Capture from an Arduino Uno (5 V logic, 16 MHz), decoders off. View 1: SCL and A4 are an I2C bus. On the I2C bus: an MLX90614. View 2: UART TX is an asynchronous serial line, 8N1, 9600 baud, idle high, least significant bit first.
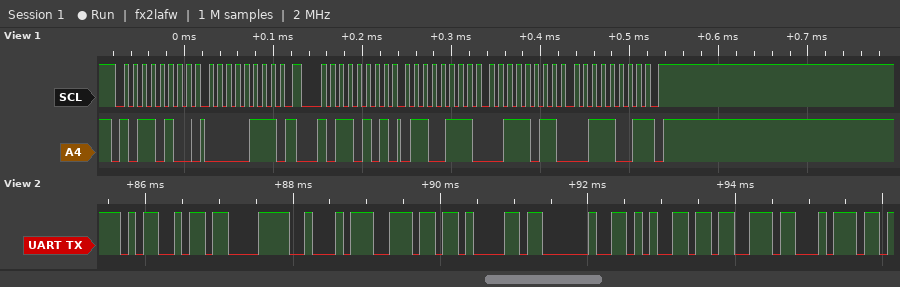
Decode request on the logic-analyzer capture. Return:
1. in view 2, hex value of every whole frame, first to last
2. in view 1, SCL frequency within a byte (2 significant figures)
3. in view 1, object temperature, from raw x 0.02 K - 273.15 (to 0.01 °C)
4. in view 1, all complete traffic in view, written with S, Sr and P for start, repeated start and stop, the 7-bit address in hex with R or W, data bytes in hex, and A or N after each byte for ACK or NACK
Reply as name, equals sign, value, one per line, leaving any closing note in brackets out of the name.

in view 2, hex value of every whole frame, first to last = 4D C3 A2 6E 61 20 65 73 74
in view 1, SCL frequency within a byte = 100 kHz
in view 1, object temperature, from raw x 0.02 K - 273.15 = 30.99 °C
in view 1, all complete traffic in view, written with S, Sr and P for start, repeated start and stop, the 7-bit address in hex with R or W, data bytes in hex, and A or N after each byte for ACK or NACK = S 5AW A 07 A Sr 5AR A 67 A 3B A 39 N P
